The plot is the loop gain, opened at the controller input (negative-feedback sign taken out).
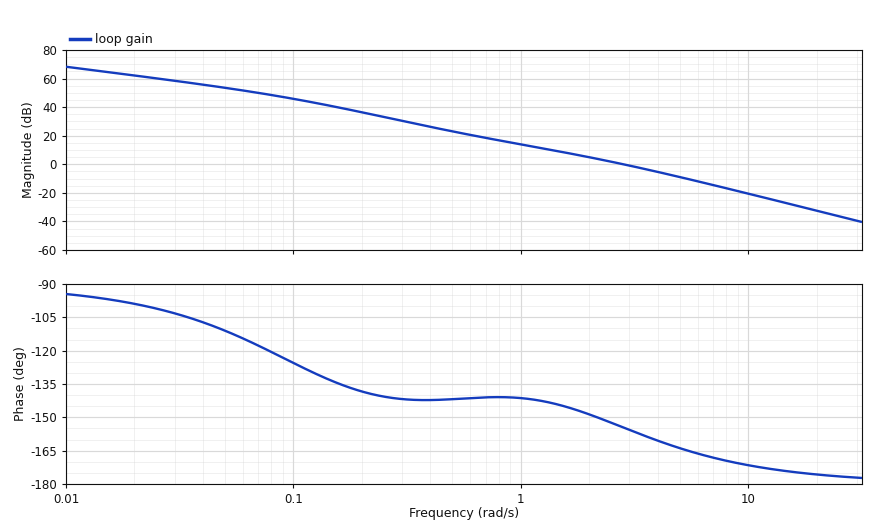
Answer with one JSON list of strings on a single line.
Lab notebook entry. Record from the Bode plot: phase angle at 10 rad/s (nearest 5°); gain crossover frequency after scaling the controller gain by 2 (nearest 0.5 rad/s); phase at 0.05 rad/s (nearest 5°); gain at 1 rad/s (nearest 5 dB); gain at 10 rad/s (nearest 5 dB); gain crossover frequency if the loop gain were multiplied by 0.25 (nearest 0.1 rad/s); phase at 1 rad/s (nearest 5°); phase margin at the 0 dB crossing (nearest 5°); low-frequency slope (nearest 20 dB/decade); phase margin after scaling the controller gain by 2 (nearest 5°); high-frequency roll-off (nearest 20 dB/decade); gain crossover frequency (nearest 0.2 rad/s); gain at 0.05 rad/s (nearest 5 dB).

["-170°", "4.0 rad/s", "-110°", "15 dB", "-20 dB", "1.2 rad/s", "-140°", "25°", "-20 dB/decade", "20°", "-40 dB/decade", "2.8 rad/s", "55 dB"]
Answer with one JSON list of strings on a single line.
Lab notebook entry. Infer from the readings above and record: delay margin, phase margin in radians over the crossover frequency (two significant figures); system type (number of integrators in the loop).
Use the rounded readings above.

["0.16 s", "1"]
